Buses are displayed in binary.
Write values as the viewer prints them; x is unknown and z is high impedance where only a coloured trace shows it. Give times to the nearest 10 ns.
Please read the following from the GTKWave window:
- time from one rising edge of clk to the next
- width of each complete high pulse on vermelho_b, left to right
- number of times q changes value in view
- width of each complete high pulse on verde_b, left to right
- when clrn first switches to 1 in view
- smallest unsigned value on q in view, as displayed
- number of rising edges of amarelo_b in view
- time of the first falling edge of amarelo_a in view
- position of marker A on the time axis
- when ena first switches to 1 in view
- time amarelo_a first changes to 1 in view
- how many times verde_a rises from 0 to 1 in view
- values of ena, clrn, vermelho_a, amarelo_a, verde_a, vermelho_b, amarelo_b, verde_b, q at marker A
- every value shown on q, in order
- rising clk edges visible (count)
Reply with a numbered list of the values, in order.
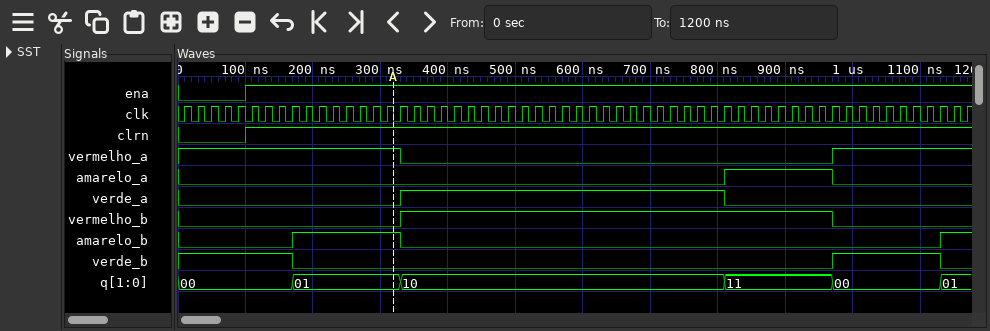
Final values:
1. 20 ns
2. 640 ns
3. 5
4. 160 ns
5. 100 ns
6. 00
7. 2
8. 970 ns
9. 320 ns
10. 100 ns
11. 810 ns
12. 1
13. ena=1, clrn=1, vermelho_a=1, amarelo_a=0, verde_a=0, vermelho_b=0, amarelo_b=1, verde_b=0, q=01
14. 00, 01, 10, 11, 00, 01
15. 59
